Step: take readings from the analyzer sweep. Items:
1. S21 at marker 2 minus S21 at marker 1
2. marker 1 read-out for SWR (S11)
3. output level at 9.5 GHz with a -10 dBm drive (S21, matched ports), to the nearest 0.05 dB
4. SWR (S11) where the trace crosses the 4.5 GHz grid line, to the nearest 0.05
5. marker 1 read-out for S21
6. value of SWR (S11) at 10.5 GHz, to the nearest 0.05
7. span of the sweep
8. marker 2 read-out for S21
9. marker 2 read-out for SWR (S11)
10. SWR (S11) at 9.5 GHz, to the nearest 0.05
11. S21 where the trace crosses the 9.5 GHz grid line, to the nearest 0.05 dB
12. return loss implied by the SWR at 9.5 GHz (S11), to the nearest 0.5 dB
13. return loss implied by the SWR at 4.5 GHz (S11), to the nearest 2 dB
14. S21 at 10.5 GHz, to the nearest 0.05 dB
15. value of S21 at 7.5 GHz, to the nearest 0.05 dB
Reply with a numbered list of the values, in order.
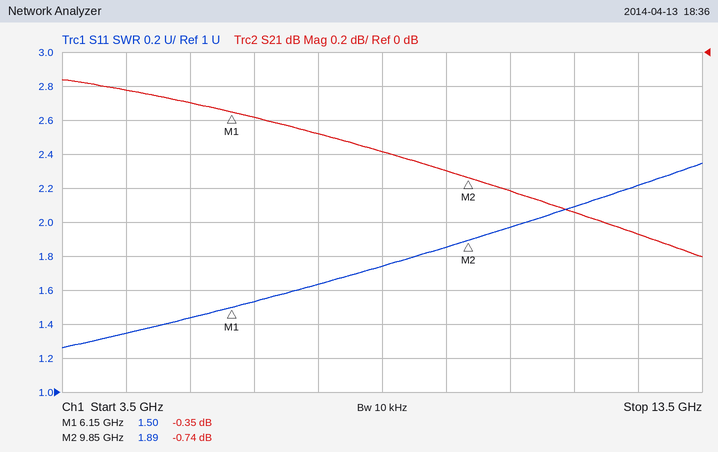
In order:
1. -0.39 dB
2. 1.50
3. -10.70 dBm
4. 1.35
5. -0.35 dB
6. 1.95
7. 10 GHz
8. -0.74 dB
9. 1.89
10. 1.85
11. -0.70 dB
12. 10.5 dB
13. 16 dB
14. -0.80 dB
15. -0.50 dB
